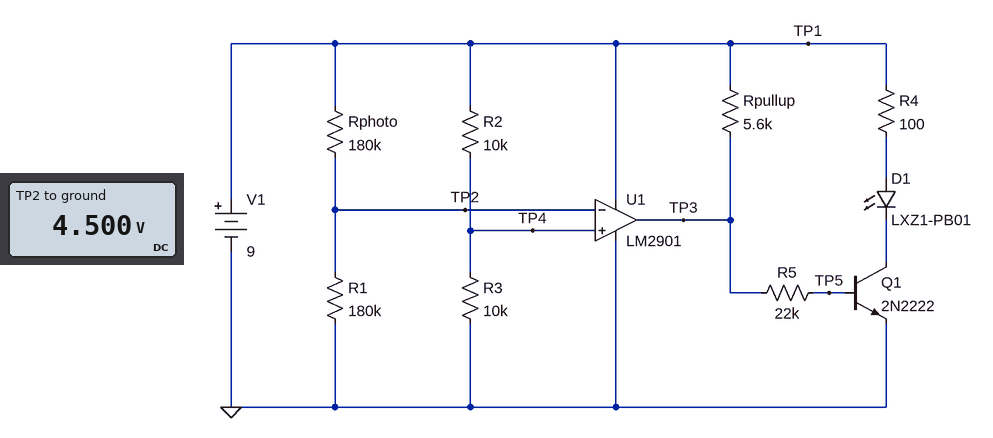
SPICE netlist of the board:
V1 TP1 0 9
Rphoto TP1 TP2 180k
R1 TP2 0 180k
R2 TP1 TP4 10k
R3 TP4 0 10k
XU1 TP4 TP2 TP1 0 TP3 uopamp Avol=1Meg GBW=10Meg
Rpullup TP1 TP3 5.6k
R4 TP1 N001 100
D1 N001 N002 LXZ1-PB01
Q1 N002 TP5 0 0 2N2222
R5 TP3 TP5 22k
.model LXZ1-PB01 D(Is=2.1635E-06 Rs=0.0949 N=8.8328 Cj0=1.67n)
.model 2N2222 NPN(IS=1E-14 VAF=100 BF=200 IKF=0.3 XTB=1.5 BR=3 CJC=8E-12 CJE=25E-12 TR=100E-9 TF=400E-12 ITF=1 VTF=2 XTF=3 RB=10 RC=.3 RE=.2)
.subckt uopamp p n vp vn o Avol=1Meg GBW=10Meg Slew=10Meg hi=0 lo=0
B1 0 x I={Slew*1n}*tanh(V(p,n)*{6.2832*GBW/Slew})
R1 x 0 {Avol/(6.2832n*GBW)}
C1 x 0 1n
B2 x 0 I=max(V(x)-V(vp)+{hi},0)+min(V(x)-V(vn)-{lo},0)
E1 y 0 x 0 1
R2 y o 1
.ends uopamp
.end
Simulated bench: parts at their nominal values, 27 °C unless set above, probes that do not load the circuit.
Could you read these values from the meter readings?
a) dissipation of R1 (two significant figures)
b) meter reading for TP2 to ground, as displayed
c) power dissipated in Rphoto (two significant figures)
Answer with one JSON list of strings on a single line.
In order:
["110 µW", "4.500 V", "110 µW"]
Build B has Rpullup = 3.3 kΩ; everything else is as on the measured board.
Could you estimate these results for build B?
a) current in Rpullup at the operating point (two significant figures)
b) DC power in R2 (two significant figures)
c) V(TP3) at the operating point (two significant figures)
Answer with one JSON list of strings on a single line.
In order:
["2.7 mA", "2.0 mW", "2.7 mV"]
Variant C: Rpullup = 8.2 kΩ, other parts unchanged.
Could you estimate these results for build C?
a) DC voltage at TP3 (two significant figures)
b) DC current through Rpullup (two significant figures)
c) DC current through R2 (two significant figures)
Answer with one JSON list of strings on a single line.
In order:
["1.1 mV", "1.1 mA", "450 µA"]
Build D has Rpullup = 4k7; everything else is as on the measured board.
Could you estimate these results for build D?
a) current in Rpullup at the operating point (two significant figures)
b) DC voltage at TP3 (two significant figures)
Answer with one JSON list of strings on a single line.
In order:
["1.9 mA", "1.9 mV"]
